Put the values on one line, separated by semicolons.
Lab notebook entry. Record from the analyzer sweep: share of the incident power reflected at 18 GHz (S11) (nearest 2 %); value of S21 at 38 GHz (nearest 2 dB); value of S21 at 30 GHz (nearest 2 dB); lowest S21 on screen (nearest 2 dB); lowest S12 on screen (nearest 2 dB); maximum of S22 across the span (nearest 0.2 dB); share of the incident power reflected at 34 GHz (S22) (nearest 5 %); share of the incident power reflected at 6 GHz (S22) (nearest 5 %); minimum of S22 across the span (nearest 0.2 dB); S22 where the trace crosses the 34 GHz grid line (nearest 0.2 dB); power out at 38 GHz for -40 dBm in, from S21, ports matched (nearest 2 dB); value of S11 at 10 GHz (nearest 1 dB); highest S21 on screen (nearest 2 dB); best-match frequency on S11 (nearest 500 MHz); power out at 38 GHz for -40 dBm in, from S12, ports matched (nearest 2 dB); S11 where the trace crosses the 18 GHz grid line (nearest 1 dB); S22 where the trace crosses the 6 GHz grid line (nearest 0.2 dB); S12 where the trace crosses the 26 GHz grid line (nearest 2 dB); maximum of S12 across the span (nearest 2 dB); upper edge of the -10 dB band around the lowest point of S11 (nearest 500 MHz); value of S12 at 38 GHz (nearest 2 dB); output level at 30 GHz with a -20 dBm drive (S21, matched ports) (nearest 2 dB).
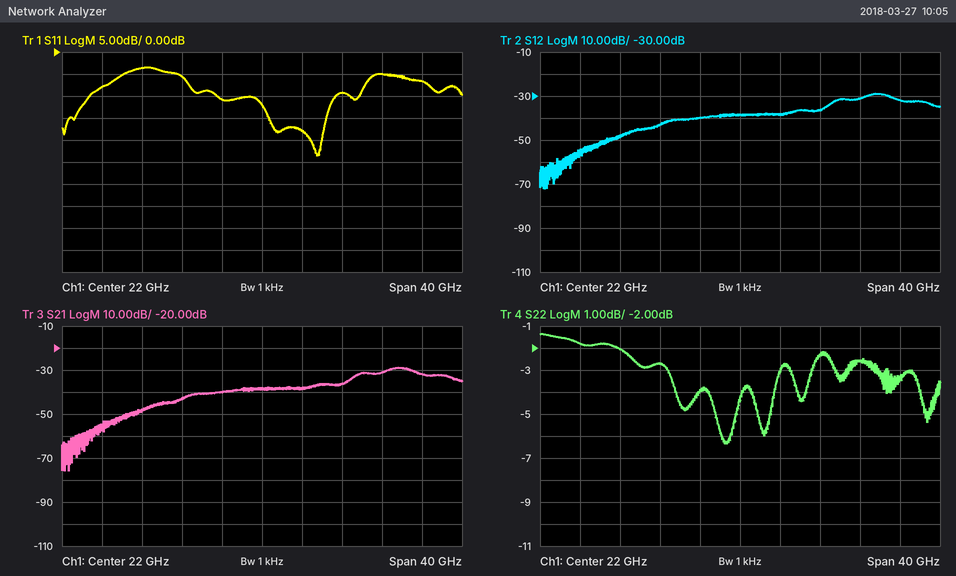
8 %; -32 dB; -36 dB; -76 dB; -72 dB; -1.4 dB; 55 %; 65 %; -6.4 dB; -2.6 dB; -72 dBm; -4 dB; -28 dB; 27.5 GHz; -72 dBm; -11 dB; -1.8 dB; -38 dB; -28 dB; 29.5 GHz; -32 dB; -56 dBm
